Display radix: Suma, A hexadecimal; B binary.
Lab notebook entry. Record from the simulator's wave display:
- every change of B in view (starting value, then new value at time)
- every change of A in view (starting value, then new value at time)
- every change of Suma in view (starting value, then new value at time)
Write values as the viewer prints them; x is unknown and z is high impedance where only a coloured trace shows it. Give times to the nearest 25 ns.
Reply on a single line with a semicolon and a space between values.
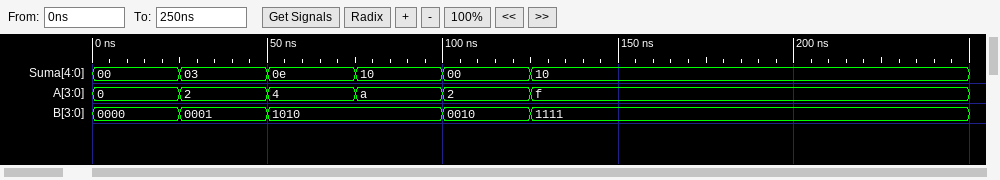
0000, 0001 at 25 ns, 1010 at 50 ns, 0010 at 100 ns, 1111 at 125 ns; 0, 2 at 25 ns, 4 at 50 ns, a at 75 ns, 2 at 100 ns, f at 125 ns; 00, 03 at 25 ns, 0e at 50 ns, 10 at 75 ns, 00 at 100 ns, 10 at 125 ns
